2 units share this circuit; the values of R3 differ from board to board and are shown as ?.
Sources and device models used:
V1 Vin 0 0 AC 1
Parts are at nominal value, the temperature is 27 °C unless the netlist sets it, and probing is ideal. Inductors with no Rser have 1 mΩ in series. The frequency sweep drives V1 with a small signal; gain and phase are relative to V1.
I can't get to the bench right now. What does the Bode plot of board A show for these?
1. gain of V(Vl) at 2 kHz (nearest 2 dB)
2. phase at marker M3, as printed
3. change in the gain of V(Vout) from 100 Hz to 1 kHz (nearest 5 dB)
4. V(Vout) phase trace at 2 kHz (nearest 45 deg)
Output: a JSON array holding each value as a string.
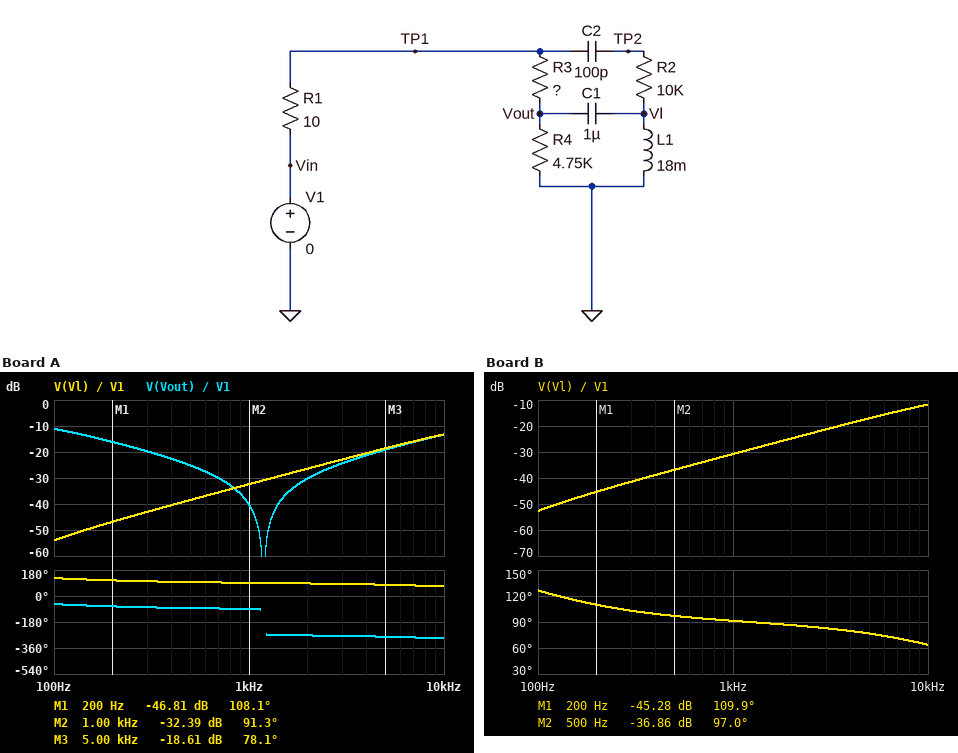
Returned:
["-26 dB", "78.1 deg", "-30 dB", "-270 deg"]
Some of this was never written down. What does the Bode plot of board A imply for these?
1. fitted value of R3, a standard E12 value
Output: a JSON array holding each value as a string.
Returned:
["4.7 kΩ"]
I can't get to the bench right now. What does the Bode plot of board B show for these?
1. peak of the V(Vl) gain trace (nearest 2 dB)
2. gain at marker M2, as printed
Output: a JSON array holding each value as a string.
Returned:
["-12 dB", "-36.86 dB"]
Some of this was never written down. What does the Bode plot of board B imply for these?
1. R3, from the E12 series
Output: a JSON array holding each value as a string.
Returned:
["3.9 kΩ"]
